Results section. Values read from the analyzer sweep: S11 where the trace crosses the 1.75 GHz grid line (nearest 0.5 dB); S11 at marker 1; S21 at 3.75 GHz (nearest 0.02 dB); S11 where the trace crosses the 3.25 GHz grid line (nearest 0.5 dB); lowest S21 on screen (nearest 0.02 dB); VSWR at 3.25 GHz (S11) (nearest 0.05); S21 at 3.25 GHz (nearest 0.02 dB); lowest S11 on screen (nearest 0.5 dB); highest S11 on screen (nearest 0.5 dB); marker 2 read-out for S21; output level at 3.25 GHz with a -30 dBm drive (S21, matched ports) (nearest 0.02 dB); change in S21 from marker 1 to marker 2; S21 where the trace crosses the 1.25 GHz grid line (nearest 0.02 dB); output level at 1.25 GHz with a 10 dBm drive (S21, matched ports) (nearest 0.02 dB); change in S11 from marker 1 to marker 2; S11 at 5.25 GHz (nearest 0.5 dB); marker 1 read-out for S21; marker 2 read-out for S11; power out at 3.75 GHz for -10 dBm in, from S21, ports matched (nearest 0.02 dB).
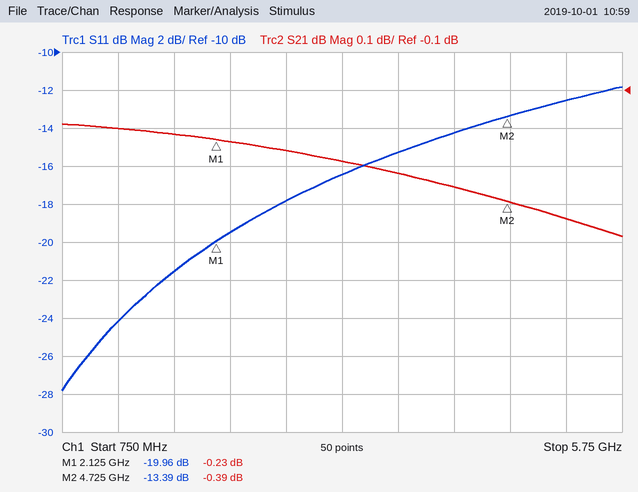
-21.5 dB
-19.96 dB
-0.32 dB
-16.5 dB
-0.48 dB
1.35
-0.28 dB
-28.0 dB
-12.0 dB
-0.39 dB
-30.28 dBm
-0.16 dB
-0.20 dB
9.80 dBm
6.57 dB
-12.5 dB
-0.23 dB
-13.39 dB
-10.32 dBm
